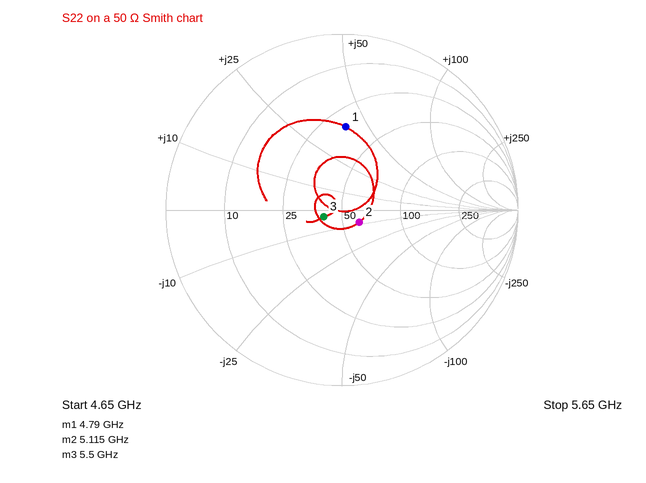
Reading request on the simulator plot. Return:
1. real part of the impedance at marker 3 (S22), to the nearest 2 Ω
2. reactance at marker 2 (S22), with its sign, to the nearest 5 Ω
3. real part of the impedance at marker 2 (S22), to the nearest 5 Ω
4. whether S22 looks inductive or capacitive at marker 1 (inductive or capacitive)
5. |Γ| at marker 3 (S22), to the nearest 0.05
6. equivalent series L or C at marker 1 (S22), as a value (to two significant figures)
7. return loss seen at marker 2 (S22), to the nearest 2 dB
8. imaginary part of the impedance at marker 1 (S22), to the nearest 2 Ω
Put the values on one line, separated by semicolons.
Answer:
40 Ω; -10 Ω; 60 Ω; inductive; 0.10; 1.3 nH; 18 dB; +40 Ω
